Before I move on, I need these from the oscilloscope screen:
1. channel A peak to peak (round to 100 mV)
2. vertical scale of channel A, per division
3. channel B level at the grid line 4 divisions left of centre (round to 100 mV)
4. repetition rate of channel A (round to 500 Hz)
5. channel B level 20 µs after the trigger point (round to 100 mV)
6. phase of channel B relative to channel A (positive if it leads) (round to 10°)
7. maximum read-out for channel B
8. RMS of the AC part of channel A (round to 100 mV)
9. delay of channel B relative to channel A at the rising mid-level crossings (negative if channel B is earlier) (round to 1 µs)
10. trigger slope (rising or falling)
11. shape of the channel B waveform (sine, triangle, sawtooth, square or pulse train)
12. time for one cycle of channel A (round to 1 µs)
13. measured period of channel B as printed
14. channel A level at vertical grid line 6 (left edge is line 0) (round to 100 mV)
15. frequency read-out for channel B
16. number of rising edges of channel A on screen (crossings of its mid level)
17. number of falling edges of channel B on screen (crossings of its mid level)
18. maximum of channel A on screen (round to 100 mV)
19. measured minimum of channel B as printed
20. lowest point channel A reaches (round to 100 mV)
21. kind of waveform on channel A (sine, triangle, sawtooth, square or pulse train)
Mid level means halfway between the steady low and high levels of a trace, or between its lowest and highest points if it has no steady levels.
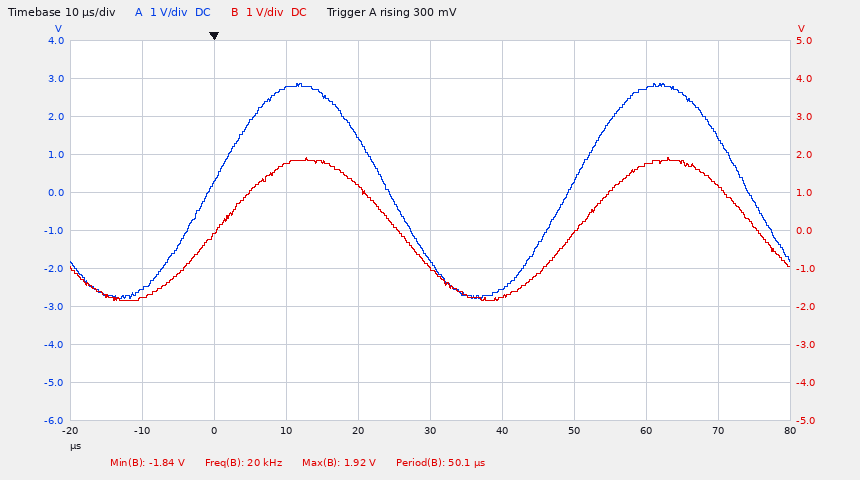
5.7 V
1 V
-1.8 V
20.0 kHz
1.2 V
-10°
1.92 V
2.0 V
+1 µs
rising
sine
50 µs
50.1 µs
-2.5 V
20 kHz
2
2
2.9 V
-1.84 V
-2.8 V
sine
